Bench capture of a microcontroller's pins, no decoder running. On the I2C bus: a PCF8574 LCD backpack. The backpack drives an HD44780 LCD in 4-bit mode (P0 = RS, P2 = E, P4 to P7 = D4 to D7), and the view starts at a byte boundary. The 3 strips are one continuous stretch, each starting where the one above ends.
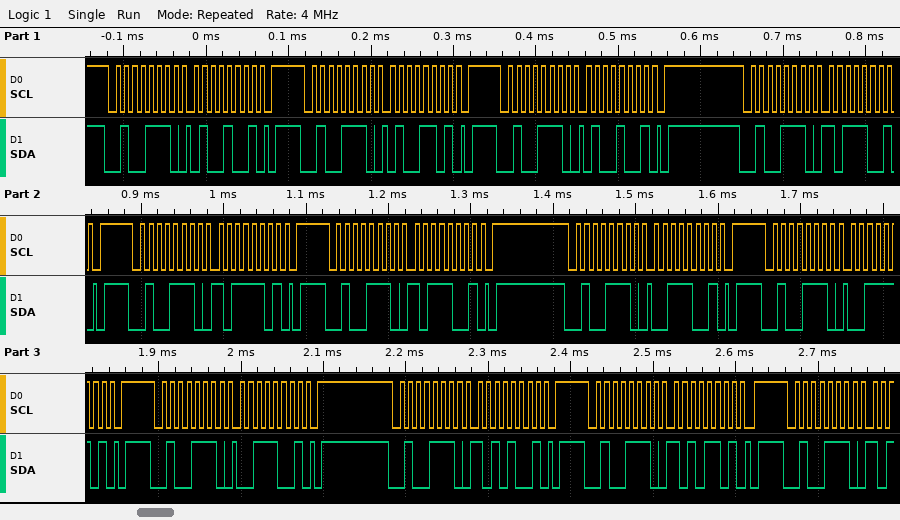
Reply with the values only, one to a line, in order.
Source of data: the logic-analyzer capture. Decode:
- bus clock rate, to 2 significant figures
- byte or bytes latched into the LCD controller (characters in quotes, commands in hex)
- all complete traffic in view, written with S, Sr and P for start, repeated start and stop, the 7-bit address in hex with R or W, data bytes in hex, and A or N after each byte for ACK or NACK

100 kHz
'K'
S 27W A 49 A P S 27W A 4D A P S 27W A 49 A P S 27W A B9 A P S 27W A BD A P S 27W A B9 A P S 27W A 39 A P S 27W A 3D A P S 27W A 39 A P S 27W A A9 A P S 27W A AD A P S 27W A
